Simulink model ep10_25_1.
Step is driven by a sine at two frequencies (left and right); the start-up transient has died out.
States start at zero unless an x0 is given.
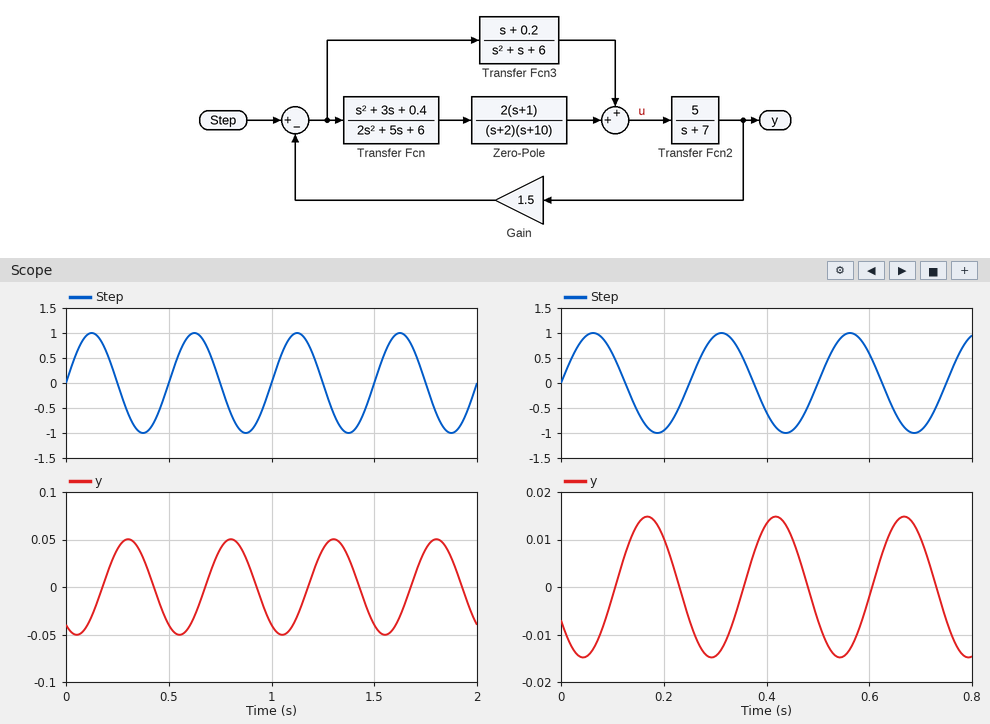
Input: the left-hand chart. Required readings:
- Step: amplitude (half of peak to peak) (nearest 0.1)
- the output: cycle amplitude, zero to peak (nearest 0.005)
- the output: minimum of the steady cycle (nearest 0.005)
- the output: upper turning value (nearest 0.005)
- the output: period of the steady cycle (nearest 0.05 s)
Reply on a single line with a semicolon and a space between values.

1.0; 0.050; -0.050; 0.050; 0.50 s
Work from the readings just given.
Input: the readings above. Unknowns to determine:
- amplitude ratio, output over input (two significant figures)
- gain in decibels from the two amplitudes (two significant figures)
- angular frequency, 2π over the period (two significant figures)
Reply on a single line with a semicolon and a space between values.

0.050; -26 dB; 13 rad/s
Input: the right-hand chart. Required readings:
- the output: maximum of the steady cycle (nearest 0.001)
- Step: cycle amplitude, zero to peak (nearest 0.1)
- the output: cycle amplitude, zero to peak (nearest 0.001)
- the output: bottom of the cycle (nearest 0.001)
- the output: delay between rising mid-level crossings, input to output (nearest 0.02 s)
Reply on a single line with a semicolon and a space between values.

0.015; 1.0; 0.015; -0.015; 0.10 s
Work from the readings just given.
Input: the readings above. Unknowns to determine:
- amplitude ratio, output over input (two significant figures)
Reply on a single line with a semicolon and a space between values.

0.015
